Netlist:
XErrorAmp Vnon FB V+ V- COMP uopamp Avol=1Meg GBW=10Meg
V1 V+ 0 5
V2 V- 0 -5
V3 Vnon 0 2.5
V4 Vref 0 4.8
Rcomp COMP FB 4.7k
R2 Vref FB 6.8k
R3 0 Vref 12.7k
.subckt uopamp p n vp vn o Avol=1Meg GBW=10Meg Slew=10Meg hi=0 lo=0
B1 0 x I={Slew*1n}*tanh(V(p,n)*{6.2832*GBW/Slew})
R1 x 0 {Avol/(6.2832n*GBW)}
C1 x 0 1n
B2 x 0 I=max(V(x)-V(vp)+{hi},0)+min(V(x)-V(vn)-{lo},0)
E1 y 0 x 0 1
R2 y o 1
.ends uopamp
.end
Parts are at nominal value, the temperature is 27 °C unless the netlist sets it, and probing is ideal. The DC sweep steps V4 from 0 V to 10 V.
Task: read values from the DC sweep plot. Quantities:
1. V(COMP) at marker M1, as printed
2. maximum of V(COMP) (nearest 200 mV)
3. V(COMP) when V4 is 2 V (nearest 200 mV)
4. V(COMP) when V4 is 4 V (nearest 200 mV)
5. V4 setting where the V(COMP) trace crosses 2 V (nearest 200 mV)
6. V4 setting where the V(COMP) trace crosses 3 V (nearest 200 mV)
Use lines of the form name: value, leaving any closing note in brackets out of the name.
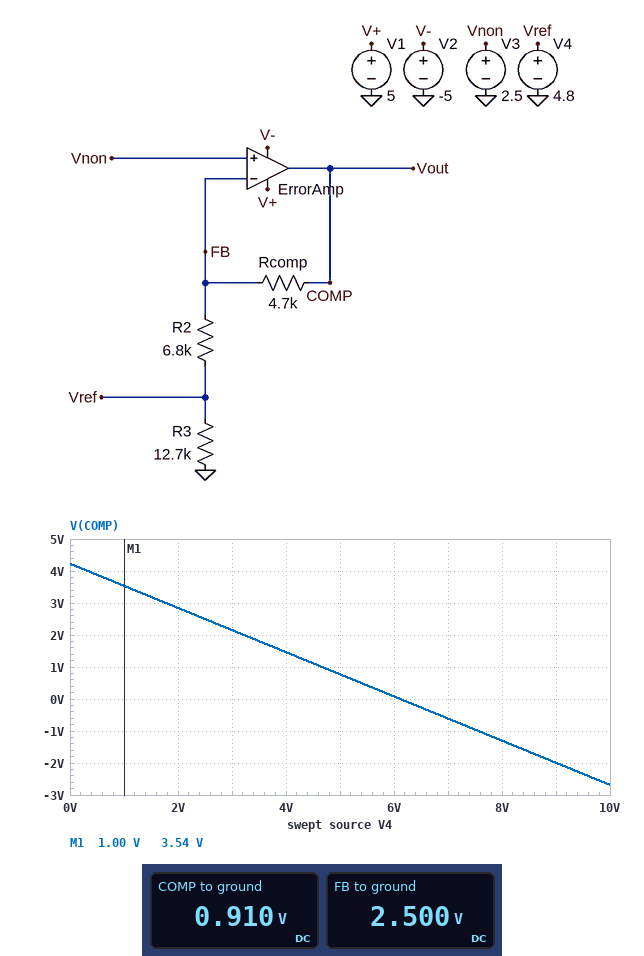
V(COMP) at marker M1, as printed: 3.54 V
maximum of V(COMP): 4.2 V
V(COMP) when V4 is 2 V: 2.8 V
V(COMP) when V4 is 4 V: 1.4 V
V4 setting where the V(COMP) trace crosses 2 V: 3.2 V
V4 setting where the V(COMP) trace crosses 3 V: 1.8 V
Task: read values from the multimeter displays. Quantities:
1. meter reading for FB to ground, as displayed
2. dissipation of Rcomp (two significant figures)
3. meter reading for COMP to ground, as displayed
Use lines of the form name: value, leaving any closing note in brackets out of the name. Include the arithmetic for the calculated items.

meter reading for FB to ground, as displayed: 2.500 V
dissipation of Rcomp: (2.5 V - 910 mV)^2 / 4.7 kΩ = 540 µW
meter reading for COMP to ground, as displayed: 0.910 V
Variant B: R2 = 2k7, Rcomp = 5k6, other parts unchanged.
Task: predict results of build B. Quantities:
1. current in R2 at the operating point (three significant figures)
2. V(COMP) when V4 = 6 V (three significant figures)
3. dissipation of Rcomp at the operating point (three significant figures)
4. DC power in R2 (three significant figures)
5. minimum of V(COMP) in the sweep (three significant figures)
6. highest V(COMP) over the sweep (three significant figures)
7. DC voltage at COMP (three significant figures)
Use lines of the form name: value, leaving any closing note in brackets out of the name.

current in R2 at the operating point: 852 µA
V(COMP) when V4 = 6 V: -4.76 V
dissipation of Rcomp at the operating point: 4.06 mW
DC power in R2: 1.96 mW
minimum of V(COMP) in the sweep: -5.01 V
highest V(COMP) over the sweep: 5.01 V
DC voltage at COMP: -2.27 V
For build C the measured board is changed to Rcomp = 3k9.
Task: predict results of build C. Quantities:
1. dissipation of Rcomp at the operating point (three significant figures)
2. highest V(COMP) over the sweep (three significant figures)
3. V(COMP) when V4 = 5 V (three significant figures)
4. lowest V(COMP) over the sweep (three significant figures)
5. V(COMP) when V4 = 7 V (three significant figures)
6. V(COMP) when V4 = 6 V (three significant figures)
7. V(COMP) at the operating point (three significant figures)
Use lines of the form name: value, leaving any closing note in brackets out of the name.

dissipation of Rcomp at the operating point: 446 µW
highest V(COMP) over the sweep: 3.93 V
V(COMP) when V4 = 5 V: 1.07 V
lowest V(COMP) over the sweep: -1.80 V
V(COMP) when V4 = 7 V: -80.9 mV
V(COMP) when V4 = 6 V: 493 mV
V(COMP) at the operating point: 1.18 V
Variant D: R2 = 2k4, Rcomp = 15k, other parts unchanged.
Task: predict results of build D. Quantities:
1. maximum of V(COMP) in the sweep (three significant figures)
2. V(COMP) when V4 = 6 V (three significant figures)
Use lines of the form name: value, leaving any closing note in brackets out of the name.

maximum of V(COMP) in the sweep: 5.01 V
V(COMP) when V4 = 6 V: -5.01 V
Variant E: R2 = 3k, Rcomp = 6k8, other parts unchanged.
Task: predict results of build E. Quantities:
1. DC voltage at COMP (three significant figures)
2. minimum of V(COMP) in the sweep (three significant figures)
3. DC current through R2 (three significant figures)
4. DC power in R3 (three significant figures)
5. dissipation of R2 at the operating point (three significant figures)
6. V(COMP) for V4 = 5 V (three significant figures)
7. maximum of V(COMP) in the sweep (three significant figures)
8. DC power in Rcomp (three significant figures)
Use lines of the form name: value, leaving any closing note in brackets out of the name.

DC voltage at COMP: -2.71 V
minimum of V(COMP) in the sweep: -5.01 V
DC current through R2: 767 µA
DC power in R3: 1.81 mW
dissipation of R2 at the operating point: 1.76 mW
V(COMP) for V4 = 5 V: -3.17 V
maximum of V(COMP) in the sweep: 5.01 V
DC power in Rcomp: 4.00 mW
